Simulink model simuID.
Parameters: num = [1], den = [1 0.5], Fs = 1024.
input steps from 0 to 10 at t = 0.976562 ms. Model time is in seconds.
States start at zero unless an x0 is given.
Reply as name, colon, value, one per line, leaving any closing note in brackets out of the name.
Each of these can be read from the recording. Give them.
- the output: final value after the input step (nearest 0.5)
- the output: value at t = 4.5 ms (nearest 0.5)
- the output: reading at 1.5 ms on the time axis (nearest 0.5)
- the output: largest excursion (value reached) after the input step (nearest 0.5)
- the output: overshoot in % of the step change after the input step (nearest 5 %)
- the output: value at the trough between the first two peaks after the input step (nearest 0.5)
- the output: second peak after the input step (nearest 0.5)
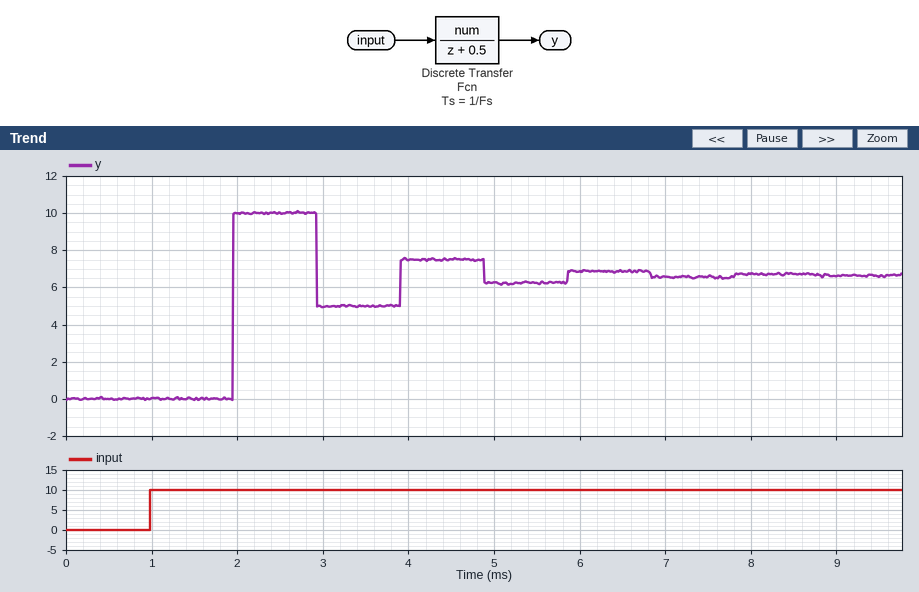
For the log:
the output: final value after the input step: 6.5
the output: value at t = 4.5 ms: 7.5
the output: reading at 1.5 ms on the time axis: 0.0
the output: largest excursion (value reached) after the input step: 10.0
the output: overshoot in % of the step change after the input step: 50 %
the output: value at the trough between the first two peaks after the input step: 5.0
the output: second peak after the input step: 7.5
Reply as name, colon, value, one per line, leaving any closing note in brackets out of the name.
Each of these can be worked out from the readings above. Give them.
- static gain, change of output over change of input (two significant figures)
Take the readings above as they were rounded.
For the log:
static gain, change of output over change of input: 0.65
